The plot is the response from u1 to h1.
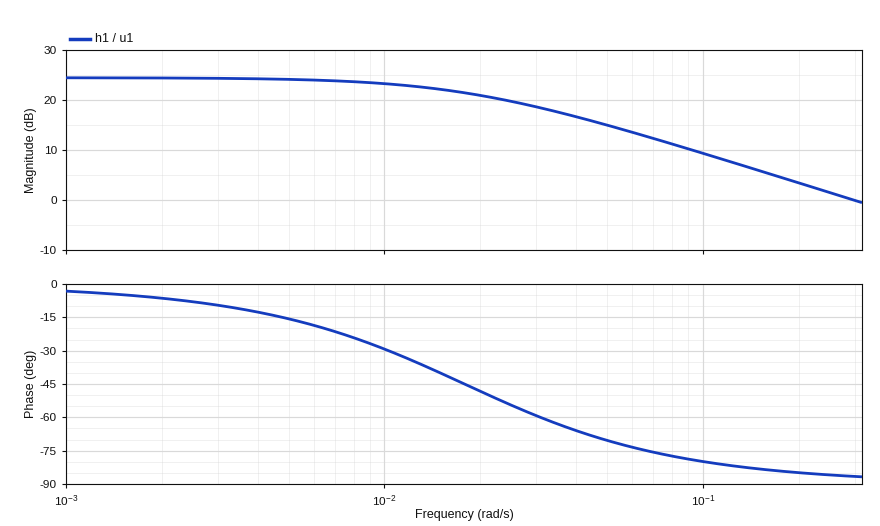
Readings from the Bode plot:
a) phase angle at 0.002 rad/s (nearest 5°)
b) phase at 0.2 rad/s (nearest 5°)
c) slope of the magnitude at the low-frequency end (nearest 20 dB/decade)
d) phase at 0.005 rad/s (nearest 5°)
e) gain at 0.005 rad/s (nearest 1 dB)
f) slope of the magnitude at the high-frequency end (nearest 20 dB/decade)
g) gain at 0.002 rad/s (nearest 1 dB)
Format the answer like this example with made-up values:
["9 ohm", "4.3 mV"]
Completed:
["-5°", "-85°", "0 dB/decade", "-15°", "24 dB", "-20 dB/decade", "24 dB"]
